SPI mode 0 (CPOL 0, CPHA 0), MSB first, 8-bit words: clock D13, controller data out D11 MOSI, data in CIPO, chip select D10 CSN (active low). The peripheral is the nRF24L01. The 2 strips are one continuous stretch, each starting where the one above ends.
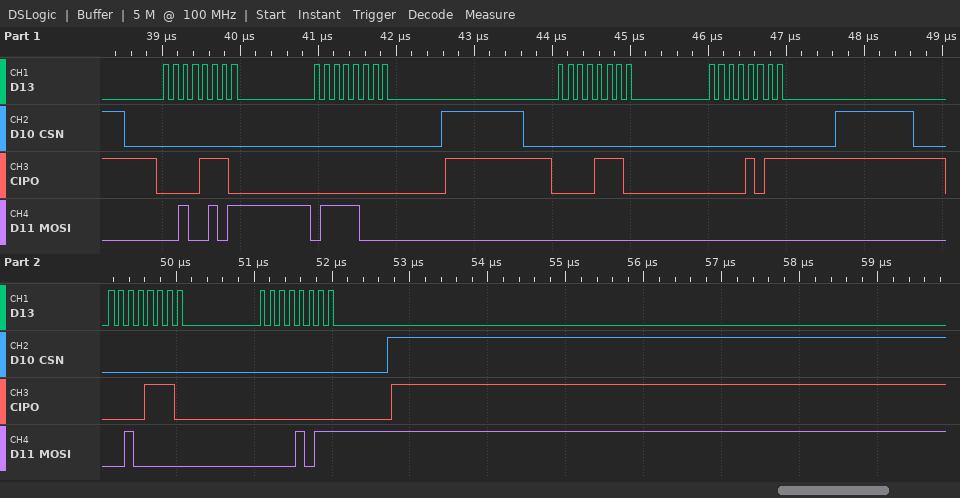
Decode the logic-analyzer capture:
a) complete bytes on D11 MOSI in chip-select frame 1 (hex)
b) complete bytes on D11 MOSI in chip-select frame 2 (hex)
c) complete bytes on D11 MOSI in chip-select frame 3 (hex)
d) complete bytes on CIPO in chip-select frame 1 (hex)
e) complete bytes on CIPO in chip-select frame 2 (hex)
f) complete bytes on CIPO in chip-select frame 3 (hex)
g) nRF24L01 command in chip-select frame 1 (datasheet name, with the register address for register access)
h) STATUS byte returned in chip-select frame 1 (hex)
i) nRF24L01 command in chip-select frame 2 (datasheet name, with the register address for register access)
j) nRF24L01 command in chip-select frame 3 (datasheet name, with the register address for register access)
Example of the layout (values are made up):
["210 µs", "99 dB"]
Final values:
["25 78", "00 00", "20 0B", "0E 00", "0E 0B", "0E 00", "W_REGISTER 0x05", "0x0E", "R_REGISTER 0x00", "W_REGISTER 0x00"]
